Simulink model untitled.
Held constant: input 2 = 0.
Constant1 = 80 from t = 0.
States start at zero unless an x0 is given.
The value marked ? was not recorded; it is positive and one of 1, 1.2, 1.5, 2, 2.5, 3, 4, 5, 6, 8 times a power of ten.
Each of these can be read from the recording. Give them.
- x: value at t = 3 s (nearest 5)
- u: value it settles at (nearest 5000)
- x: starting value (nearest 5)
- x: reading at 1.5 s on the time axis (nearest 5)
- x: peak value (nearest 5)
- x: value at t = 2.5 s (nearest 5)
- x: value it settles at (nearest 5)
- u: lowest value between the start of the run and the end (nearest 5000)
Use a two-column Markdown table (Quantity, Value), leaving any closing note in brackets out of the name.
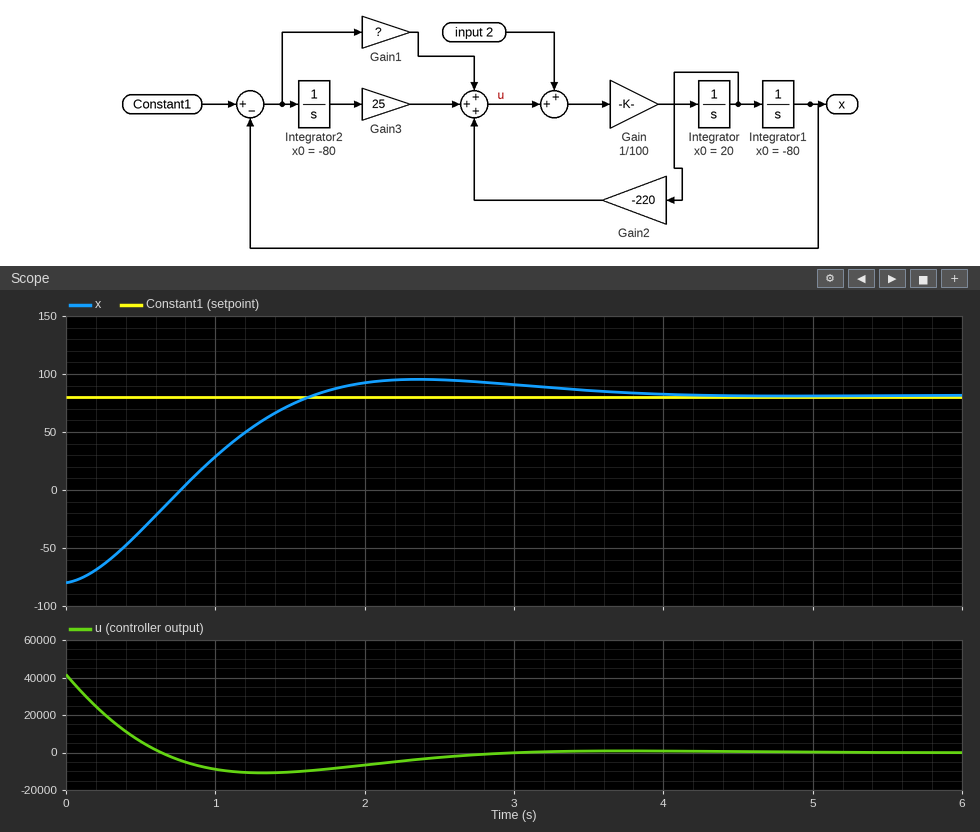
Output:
| Quantity | Value |
|---|---|
| x: value at t = 3 s | 90 |
| u: value it settles at | 0 |
| x: starting value | -80 |
| x: reading at 1.5 s on the time axis | 75 |
| x: peak value | 95 |
| x: value at t = 2.5 s | 95 |
| x: value it settles at | 80 |
| u: lowest value between the start of the run and the end | -10000 |
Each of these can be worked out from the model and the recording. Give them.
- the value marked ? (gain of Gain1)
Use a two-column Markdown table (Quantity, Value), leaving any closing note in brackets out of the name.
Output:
| Quantity | Value |
|---|---|
| the value marked ? | 300 |
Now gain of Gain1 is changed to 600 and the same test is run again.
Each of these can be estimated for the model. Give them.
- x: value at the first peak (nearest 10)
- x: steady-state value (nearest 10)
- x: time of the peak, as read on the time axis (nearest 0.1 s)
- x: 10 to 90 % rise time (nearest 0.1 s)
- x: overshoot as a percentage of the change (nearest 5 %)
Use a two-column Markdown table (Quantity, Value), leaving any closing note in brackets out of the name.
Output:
| Quantity | Value |
|---|---|
| x: value at the first peak | 110 |
| x: steady-state value | 80 |
| x: time of the peak, as read on the time axis | 1.4 s |
| x: 10 to 90 % rise time | 0.6 s |
| x: overshoot as a percentage of the change | 20 % |
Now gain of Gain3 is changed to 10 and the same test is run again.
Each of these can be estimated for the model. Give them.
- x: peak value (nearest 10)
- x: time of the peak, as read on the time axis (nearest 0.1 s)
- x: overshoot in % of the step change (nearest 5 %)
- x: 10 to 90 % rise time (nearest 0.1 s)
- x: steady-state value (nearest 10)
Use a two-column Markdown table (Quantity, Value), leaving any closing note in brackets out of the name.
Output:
| Quantity | Value |
|---|---|
| x: peak value | 90 |
| x: time of the peak, as read on the time axis | 2.3 s |
| x: overshoot in % of the step change | 10 % |
| x: 10 to 90 % rise time | 1.1 s |
| x: steady-state value | 80 |
